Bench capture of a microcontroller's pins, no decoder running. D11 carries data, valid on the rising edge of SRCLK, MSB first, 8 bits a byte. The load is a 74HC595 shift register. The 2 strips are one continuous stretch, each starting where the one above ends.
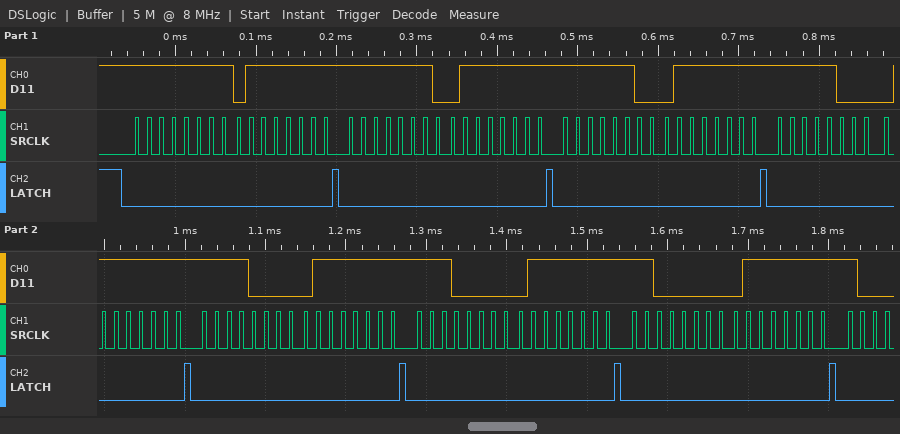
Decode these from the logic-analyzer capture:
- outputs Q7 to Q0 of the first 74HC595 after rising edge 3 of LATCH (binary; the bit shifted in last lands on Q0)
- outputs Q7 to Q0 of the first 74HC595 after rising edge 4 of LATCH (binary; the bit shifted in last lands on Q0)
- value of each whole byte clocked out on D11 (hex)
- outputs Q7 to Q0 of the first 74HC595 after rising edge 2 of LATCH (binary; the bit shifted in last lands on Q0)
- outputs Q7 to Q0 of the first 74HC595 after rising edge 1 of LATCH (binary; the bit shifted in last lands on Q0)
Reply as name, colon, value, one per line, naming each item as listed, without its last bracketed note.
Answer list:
outputs Q7 to Q0 of the first 74HC595 after rising edge 3 of LATCH: 01111111
outputs Q7 to Q0 of the first 74HC595 after rising edge 4 of LATCH: 01111111
value of each whole byte clocked out on D11: FF 7F FE 7F FC 7F F8 7F F0 7F E0 7F C0 7F
outputs Q7 to Q0 of the first 74HC595 after rising edge 2 of LATCH: 01111111
outputs Q7 to Q0 of the first 74HC595 after rising edge 1 of LATCH: 01111111
